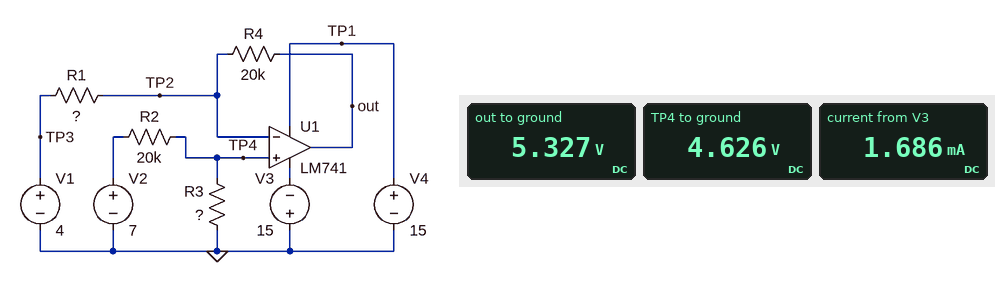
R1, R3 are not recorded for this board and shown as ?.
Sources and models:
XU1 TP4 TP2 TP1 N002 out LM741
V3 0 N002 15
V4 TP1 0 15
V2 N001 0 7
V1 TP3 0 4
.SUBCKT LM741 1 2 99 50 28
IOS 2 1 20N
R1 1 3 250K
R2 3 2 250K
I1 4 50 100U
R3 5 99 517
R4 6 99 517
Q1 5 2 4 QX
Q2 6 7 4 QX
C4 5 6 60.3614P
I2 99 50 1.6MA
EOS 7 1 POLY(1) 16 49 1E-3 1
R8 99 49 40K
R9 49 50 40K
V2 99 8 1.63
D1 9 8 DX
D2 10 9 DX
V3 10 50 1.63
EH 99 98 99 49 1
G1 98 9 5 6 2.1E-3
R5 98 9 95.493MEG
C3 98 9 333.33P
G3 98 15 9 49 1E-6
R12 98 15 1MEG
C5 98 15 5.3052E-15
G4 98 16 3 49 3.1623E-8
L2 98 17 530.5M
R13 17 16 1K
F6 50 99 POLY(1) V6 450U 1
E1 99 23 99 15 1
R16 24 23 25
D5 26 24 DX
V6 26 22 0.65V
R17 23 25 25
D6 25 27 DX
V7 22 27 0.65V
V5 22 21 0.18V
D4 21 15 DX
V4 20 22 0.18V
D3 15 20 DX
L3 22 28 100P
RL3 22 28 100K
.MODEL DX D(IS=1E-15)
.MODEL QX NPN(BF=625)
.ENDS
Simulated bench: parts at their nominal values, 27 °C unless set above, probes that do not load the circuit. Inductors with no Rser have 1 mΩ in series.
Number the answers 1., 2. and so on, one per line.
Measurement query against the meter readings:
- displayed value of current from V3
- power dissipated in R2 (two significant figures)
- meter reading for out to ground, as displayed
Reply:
1. 1.686 mA
2. 280 µW
3. 5.327 V
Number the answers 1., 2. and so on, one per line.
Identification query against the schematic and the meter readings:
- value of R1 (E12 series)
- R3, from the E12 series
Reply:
1. 18 kΩ
2. 39 kΩ
